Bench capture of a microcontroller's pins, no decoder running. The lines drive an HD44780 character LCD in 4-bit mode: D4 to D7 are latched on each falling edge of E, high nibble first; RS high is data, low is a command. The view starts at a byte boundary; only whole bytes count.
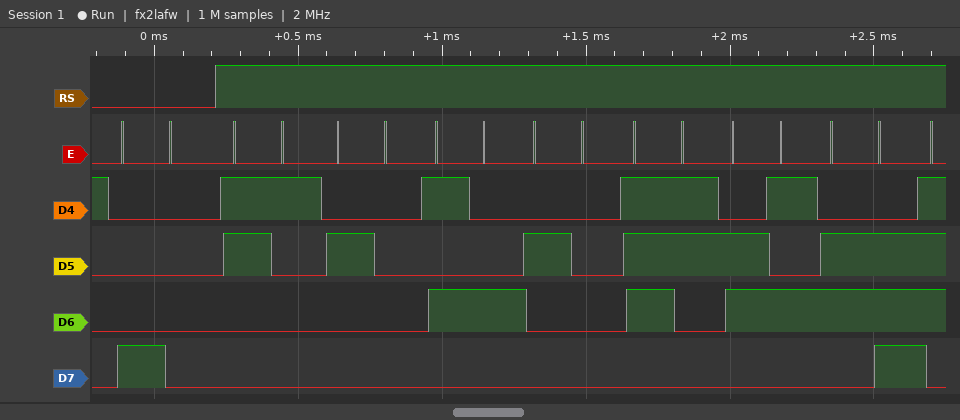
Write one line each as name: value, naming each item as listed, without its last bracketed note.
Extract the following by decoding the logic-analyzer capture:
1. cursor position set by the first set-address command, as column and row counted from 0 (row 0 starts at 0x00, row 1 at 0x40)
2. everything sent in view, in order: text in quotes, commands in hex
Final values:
cursor position set by the first set-address command, as column and row counted from 0: column 0, row 0
everything sent in view, in order: text in quotes, commands in hex: 0x80 "1 T sen"
